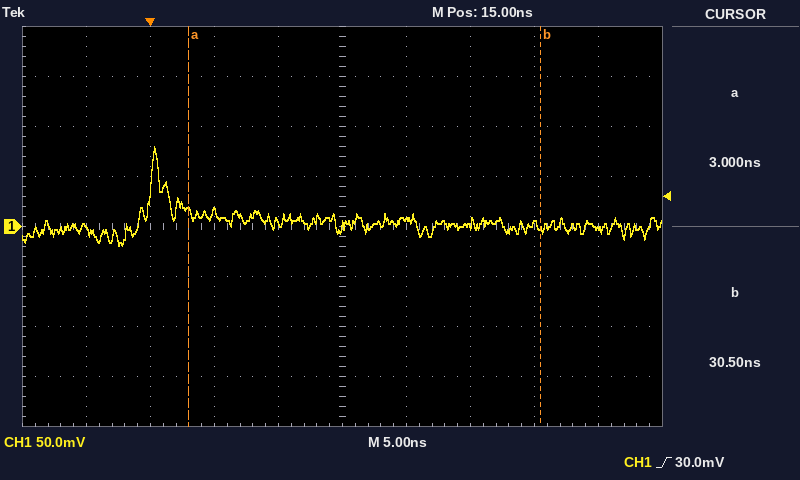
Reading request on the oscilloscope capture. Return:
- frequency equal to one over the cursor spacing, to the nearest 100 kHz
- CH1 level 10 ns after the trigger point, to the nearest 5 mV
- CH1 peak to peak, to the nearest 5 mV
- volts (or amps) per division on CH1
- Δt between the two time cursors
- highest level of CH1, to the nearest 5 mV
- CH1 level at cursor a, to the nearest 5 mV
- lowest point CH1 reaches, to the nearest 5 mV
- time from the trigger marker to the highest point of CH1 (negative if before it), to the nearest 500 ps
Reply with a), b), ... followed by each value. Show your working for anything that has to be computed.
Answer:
a) 1 / 27.5 ns ≈ 36.4 MHz
b) 5 mV
c) 80 mV − (-20 mV) = 100 mV
d) 50 mV
e) 30.5 ns − (3 ns) = 27.5 ns
f) 80 mV
g) 15 mV
h) -20 mV
i) +500 ps
